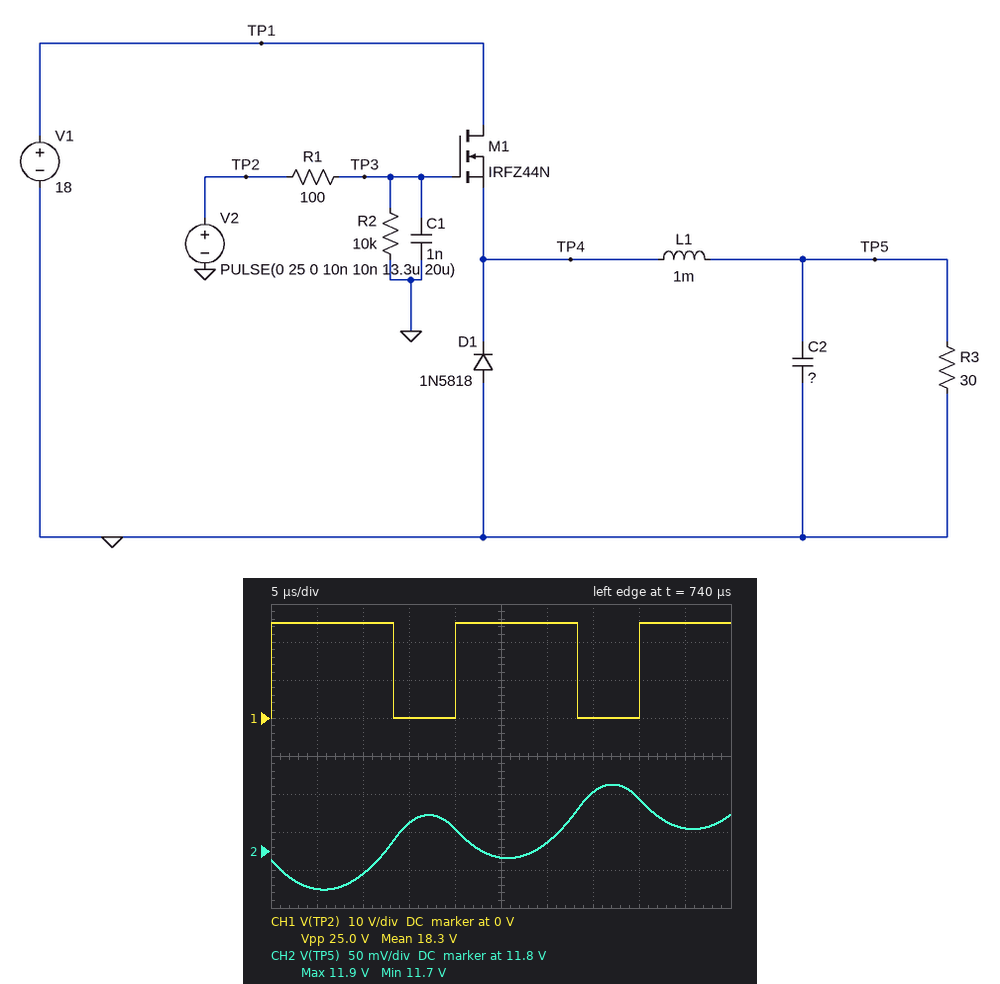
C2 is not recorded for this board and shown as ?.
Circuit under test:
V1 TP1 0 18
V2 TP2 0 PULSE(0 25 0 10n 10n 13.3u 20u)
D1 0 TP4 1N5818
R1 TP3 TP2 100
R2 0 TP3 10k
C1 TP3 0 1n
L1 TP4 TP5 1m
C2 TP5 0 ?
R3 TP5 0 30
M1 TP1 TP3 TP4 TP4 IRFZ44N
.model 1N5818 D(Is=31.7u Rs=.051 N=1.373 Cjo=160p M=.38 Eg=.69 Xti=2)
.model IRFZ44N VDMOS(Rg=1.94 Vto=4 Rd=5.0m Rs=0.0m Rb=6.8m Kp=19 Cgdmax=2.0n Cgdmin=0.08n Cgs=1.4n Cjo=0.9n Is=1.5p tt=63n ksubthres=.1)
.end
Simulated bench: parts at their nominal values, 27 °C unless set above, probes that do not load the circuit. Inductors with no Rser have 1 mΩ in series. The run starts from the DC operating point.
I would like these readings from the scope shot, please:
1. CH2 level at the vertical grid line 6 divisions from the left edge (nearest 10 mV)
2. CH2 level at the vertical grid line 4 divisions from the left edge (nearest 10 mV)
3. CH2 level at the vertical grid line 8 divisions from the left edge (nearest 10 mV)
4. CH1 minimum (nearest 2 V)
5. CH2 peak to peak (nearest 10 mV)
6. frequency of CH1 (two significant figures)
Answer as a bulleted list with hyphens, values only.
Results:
- 11.81 V
- 11.83 V
- 11.87 V
- 0 V
- 140 mV
- 50 kHz
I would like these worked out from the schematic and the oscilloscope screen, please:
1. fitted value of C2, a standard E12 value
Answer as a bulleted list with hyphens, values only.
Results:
- 2.7 µF
